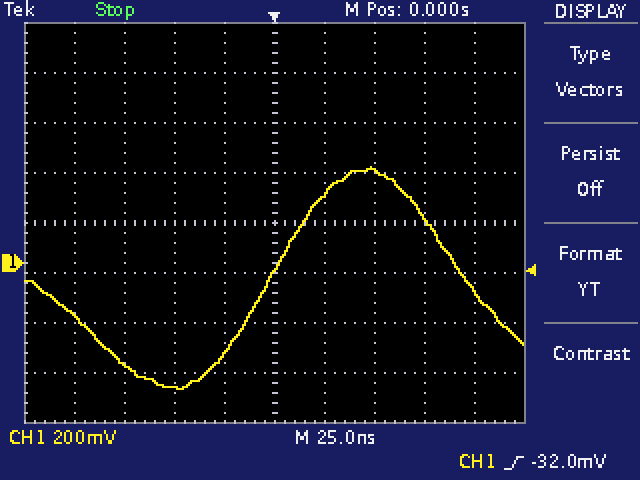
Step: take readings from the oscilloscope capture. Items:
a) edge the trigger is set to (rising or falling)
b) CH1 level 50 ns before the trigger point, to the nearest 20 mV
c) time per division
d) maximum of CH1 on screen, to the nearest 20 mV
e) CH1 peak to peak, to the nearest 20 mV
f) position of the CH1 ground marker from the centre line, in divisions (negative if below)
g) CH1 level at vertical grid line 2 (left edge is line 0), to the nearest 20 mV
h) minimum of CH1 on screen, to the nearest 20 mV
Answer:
rising
-500 mV
25 ns
380 mV
880 mV
-0.8 div
-400 mV
-500 mV
